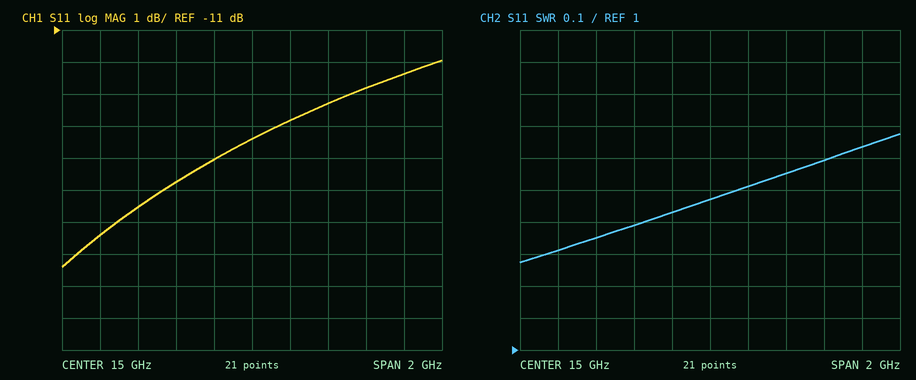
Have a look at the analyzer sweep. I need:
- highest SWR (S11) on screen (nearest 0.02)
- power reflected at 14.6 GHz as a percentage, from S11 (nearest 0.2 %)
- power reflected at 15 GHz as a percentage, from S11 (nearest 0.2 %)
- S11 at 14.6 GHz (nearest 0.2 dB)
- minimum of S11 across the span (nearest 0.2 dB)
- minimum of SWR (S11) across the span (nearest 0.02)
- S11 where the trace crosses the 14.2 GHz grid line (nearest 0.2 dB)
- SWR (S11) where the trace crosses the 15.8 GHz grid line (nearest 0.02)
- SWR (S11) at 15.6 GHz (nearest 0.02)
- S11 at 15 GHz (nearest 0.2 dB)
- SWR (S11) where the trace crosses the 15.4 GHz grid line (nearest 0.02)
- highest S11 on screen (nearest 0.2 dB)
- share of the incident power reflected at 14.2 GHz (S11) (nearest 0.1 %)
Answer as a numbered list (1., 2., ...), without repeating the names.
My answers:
1. 1.68
2. 2.6 %
3. 3.6 %
4. -15.8 dB
5. -18.4 dB
6. 1.28
7. -17.4 dB
8. 1.64
9. 1.60
10. -14.4 dB
11. 1.56
12. -12.0 dB
13. 1.8 %
